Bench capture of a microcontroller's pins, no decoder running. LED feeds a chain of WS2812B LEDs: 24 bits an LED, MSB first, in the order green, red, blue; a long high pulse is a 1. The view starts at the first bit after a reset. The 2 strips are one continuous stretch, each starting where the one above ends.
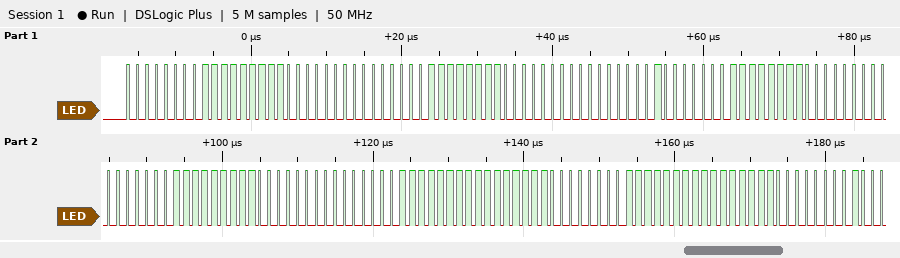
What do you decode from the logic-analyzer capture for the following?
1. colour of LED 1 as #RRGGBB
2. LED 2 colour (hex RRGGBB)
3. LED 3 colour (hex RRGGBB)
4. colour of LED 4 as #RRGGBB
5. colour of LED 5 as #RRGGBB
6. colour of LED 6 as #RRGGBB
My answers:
#FF0080
#FF0000
#8000FF
#0000FF
#0080FF
#00FFFF
